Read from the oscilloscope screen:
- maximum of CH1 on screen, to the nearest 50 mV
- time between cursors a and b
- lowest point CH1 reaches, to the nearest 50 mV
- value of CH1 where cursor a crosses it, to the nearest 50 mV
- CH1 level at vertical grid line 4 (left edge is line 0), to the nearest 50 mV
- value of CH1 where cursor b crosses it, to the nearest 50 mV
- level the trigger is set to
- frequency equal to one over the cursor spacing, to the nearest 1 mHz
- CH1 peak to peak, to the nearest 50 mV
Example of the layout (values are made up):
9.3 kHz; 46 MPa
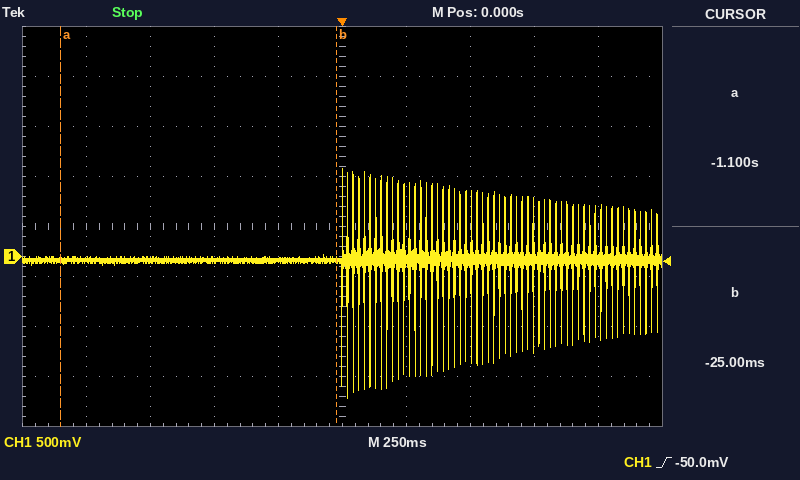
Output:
900 mV; 1.075 s; -1.40 V; -50 mV; -50 mV; -50 mV; -50.0 mV; 930 mHz; 2.30 V
